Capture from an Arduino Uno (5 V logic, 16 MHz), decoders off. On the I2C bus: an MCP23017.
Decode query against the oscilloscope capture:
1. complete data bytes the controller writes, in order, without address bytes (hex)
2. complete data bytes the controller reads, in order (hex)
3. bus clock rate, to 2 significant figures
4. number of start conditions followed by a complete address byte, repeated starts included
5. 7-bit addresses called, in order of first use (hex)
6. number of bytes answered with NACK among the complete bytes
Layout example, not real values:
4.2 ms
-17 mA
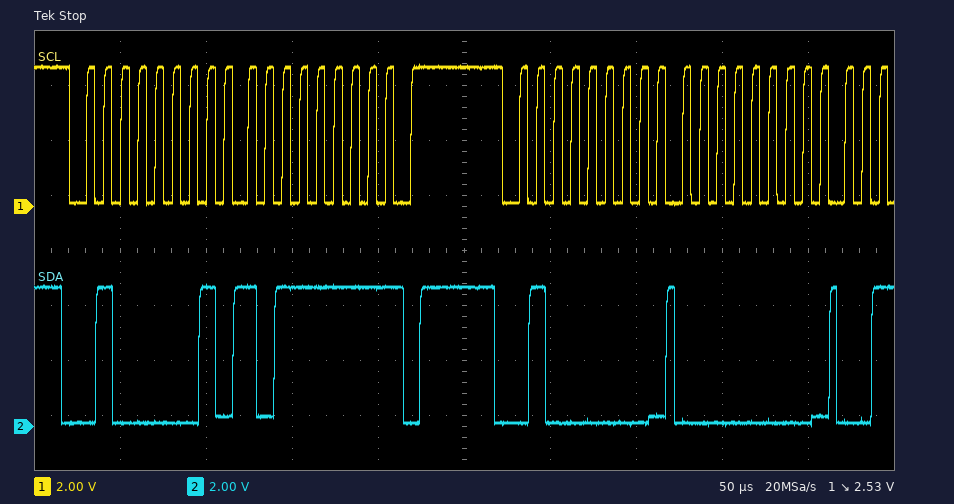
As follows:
00
BF
100 kHz
2
0x20
1
